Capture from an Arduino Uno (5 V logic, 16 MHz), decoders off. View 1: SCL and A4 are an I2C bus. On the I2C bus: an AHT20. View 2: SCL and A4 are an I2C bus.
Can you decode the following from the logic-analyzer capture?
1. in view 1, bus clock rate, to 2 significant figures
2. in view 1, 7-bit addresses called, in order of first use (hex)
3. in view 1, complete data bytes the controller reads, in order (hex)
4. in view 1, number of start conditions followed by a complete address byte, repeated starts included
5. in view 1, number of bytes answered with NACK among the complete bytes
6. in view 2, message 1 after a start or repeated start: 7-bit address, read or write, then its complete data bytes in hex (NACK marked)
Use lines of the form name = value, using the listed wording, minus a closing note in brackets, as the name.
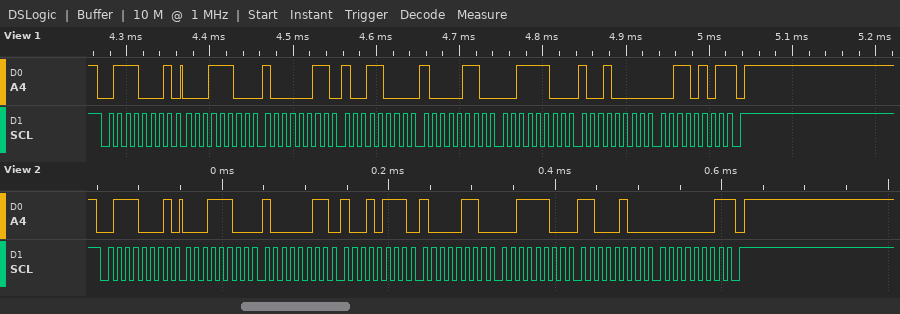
in view 1, bus clock rate, to 2 significant figures = 100 kHz
in view 1, 7-bit addresses called, in order of first use = 0x38
in view 1, complete data bytes the controller reads, in order = 1C 83 98 86 3C 90 35
in view 1, number of start conditions followed by a complete address byte, repeated starts included = 1
in view 1, number of bytes answered with NACK among the complete bytes = 1
in view 2, message 1 after a start or repeated start: 7-bit address, read or write, then its complete data bytes in hex = 0x38 read: 1C 83 97 86 3C C4 01 NACK
